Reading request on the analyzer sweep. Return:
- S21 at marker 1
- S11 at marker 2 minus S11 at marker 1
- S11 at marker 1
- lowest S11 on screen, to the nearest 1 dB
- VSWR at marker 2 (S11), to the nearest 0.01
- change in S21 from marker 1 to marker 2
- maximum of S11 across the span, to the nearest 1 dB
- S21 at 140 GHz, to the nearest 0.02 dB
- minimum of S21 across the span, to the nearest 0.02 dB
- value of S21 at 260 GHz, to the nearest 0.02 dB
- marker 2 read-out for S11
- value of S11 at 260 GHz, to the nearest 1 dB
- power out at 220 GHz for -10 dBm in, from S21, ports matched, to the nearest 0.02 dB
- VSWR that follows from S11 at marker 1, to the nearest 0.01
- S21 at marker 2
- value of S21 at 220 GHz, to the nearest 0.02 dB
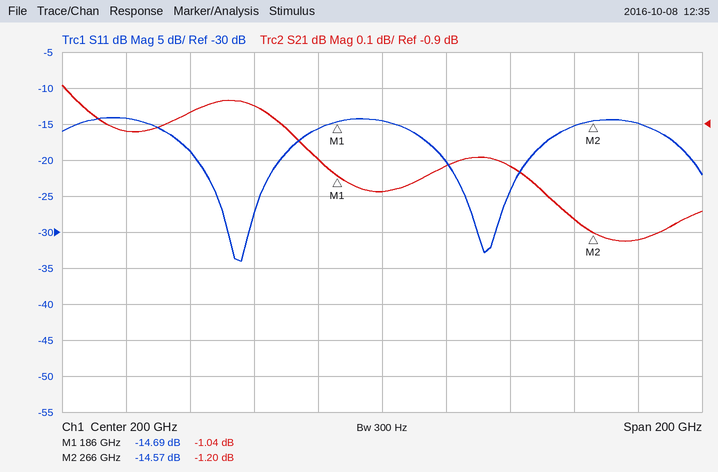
-1.04 dB
0.12 dB
-14.69 dB
-34 dB
1.46
-0.16 dB
-14 dB
-0.86 dB
-1.22 dB
-1.16 dB
-14.57 dB
-15 dB
-11.02 dBm
1.45
-1.20 dB
-1.02 dB
